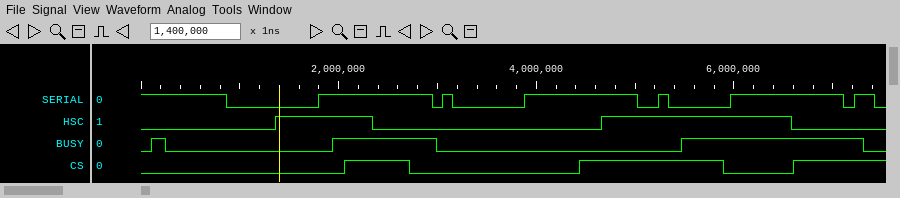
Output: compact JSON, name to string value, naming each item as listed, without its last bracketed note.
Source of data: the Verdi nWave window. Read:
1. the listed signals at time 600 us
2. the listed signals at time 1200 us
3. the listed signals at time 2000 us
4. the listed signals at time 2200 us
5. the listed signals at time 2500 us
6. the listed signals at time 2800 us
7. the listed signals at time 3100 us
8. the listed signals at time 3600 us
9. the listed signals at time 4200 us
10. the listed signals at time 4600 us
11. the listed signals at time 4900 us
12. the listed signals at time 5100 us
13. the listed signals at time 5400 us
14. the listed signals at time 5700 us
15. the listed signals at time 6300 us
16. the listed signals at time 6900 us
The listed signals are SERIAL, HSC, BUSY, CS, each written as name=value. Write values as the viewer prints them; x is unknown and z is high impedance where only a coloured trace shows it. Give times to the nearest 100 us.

{"the listed signals at time 600 us": "SERIAL=1, HSC=0, BUSY=0, CS=0", "the listed signals at time 1200 us": "SERIAL=0, HSC=0, BUSY=0, CS=0", "the listed signals at time 2000 us": "SERIAL=1, HSC=1, BUSY=1, CS=0", "the listed signals at time 2200 us": "SERIAL=1, HSC=1, BUSY=1, CS=1", "the listed signals at time 2500 us": "SERIAL=1, HSC=0, BUSY=1, CS=1", "the listed signals at time 2800 us": "SERIAL=1, HSC=0, BUSY=1, CS=0", "the listed signals at time 3100 us": "SERIAL=1, HSC=0, BUSY=0, CS=0", "the listed signals at time 3600 us": "SERIAL=0, HSC=0, BUSY=0, CS=0", "the listed signals at time 4200 us": "SERIAL=1, HSC=0, BUSY=0, CS=0", "the listed signals at time 4600 us": "SERIAL=1, HSC=0, BUSY=0, CS=1", "the listed signals at time 4900 us": "SERIAL=1, HSC=1, BUSY=0, CS=1", "the listed signals at time 5100 us": "SERIAL=0, HSC=1, BUSY=0, CS=1", "the listed signals at time 5400 us": "SERIAL=0, HSC=1, BUSY=0, CS=1", "the listed signals at time 5700 us": "SERIAL=0, HSC=1, BUSY=1, CS=1", "the listed signals at time 6300 us": "SERIAL=1, HSC=1, BUSY=1, CS=0", "the listed signals at time 6900 us": "SERIAL=1, HSC=0, BUSY=1, CS=1"}
